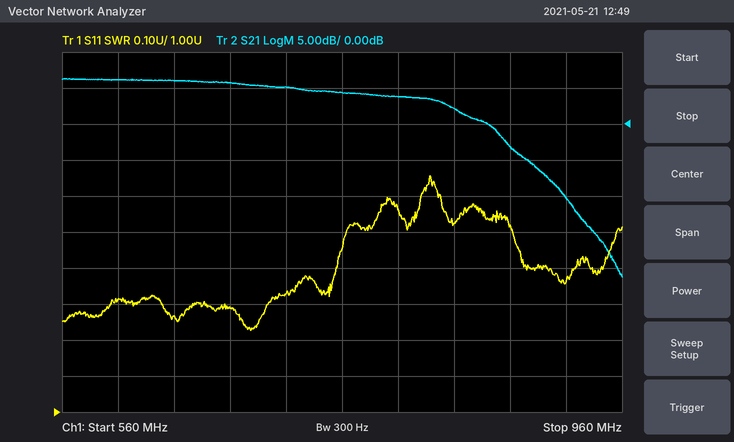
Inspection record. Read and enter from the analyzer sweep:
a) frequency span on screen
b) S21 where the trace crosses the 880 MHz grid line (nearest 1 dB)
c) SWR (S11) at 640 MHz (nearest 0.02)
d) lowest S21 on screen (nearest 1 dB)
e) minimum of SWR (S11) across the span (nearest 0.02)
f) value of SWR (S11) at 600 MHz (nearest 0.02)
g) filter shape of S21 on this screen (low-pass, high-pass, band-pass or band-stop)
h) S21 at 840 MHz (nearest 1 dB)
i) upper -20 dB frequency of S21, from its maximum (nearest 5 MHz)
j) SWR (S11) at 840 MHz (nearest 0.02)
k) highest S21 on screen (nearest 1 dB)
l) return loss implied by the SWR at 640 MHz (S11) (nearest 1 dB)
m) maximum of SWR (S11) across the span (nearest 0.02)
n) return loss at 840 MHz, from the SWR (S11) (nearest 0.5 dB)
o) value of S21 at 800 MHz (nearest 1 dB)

400 MHz
-3 dB
1.26
-21 dB
1.22
1.32
low-pass
2 dB
935 MHz
1.52
6 dB
19 dB
1.66
13.5 dB
4 dB
